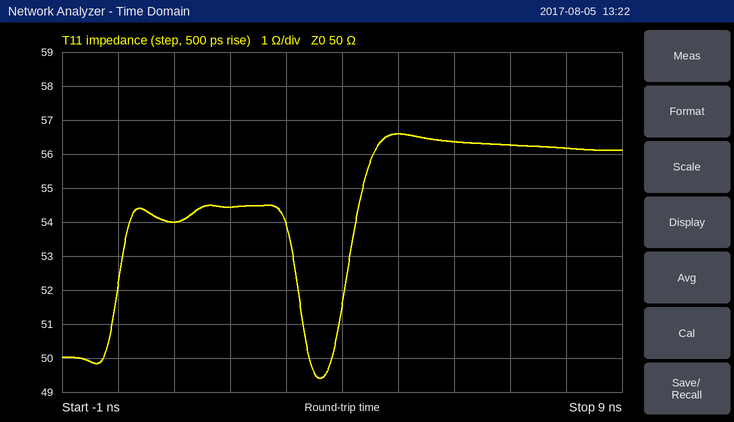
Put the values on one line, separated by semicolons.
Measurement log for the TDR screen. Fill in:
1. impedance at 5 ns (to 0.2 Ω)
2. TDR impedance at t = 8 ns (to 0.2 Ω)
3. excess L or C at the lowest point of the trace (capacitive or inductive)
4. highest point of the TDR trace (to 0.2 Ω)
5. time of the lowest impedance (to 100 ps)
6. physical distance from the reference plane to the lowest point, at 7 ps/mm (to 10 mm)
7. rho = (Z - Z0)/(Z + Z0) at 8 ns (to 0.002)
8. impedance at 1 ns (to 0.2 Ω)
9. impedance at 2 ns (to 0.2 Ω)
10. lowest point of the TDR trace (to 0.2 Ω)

56.6 Ω; 56.2 Ω; capacitive; 56.6 Ω; 3.6 ns; 260 mm; +0.058; 54.0 Ω; 54.4 Ω; 49.4 Ω
